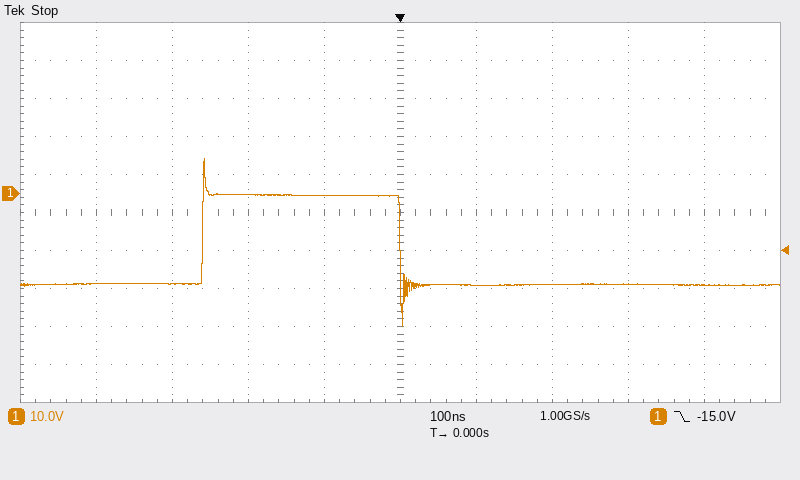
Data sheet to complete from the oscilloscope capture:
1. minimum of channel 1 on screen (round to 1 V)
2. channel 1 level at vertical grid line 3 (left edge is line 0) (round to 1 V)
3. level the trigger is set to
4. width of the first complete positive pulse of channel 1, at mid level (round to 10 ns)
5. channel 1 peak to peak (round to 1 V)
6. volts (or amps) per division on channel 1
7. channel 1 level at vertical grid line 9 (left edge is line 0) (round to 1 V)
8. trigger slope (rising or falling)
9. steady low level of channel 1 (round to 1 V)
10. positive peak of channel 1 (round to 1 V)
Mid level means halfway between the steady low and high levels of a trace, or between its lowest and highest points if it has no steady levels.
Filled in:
-35 V
0 V
-15.0 V
260 ns
44 V
10 V
-24 V
falling
-24 V
9 V
